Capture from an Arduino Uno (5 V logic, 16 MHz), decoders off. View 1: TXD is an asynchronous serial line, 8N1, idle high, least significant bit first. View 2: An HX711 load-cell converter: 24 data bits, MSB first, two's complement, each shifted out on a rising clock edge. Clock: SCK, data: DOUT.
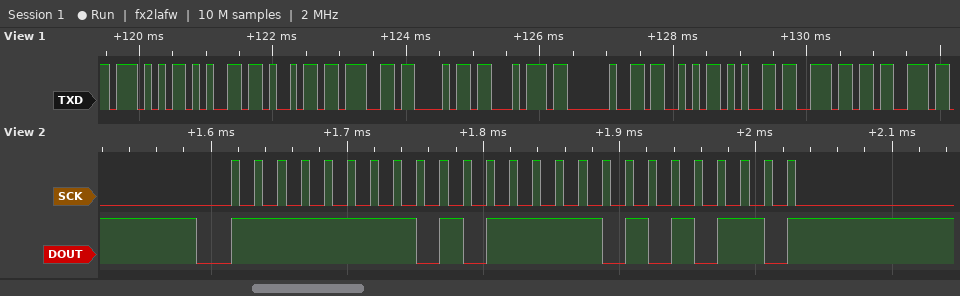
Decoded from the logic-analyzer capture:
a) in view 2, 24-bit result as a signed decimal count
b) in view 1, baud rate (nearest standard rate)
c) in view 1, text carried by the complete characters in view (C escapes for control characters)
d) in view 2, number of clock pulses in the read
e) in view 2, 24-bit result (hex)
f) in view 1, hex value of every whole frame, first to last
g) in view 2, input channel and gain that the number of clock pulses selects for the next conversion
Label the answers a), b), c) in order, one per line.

a) -41130
b) 9600 baud
c) "Weight Sens"
d) 25
e) 0xFF5F56
f) 57 65 69 67 68 74 20 53 65 6E 73
g) channel A, gain 128
